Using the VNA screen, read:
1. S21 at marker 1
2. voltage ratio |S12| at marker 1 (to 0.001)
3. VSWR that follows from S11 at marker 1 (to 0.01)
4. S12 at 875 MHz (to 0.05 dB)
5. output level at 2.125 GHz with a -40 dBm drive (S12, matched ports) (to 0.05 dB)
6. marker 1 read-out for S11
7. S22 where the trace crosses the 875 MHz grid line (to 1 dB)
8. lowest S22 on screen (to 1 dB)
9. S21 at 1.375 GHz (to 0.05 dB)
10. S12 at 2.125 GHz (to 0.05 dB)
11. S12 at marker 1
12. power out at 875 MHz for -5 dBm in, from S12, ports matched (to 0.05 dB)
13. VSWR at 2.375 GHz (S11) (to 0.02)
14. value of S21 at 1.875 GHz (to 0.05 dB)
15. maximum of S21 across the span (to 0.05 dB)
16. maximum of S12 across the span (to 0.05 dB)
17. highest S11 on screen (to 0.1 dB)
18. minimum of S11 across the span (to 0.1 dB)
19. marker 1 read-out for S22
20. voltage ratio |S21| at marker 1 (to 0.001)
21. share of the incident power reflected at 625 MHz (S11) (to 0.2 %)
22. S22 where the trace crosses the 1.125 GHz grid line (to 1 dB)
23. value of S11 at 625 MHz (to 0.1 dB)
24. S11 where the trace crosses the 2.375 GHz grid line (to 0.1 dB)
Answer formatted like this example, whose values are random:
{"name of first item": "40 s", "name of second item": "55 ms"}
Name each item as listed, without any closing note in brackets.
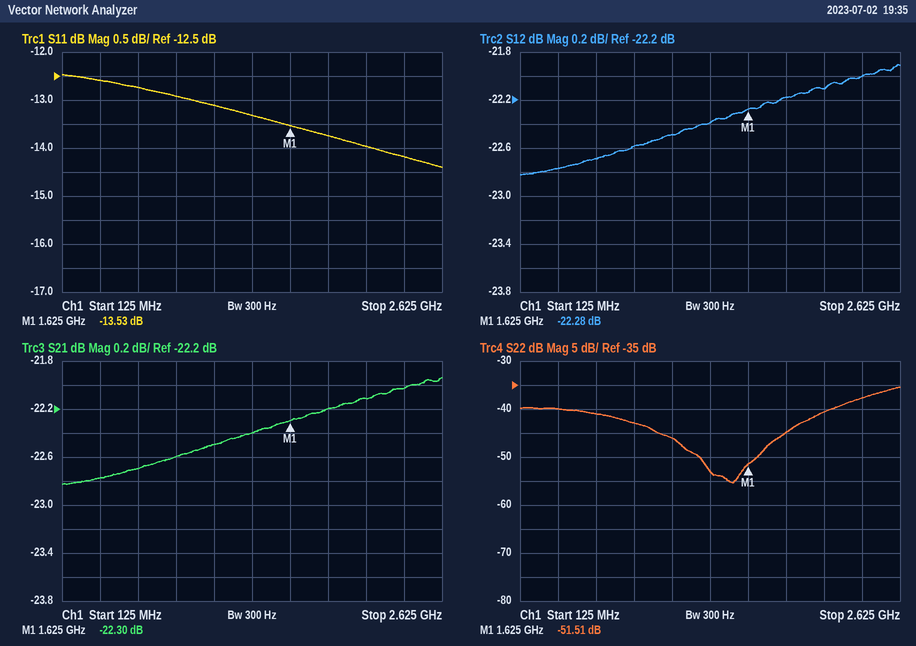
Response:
{"S21 at marker 1": "-22.30 dB", "voltage ratio |S12| at marker 1": "0.077", "VSWR that follows from S11 at marker 1": "1.53", "S12 at 875 MHz": "-22.60 dB", "output level at 2.125 GHz with a -40 dBm drive (S12, matched ports)": "-62.10 dBm", "marker 1 read-out for S11": "-13.53 dB", "S22 where the trace crosses the 875 MHz grid line": "-43 dB", "lowest S22 on screen": "-55 dB", "S21 at 1.375 GHz": "-22.40 dB", "S12 at 2.125 GHz": "-22.10 dB", "S12 at marker 1": "-22.28 dB", "power out at 875 MHz for -5 dBm in, from S12, ports matched": "-27.60 dBm", "VSWR at 2.375 GHz (S11)": "1.48", "value of S21 at 1.875 GHz": "-22.20 dB", "maximum of S21 across the span": "-21.95 dB", "maximum of S12 across the span": "-21.90 dB", "highest S11 on screen": "-12.5 dB", "minimum of S11 across the span": "-14.4 dB", "marker 1 read-out for S22": "-51.51 dB", "voltage ratio |S21| at marker 1": "0.077", "share of the incident power reflected at 625 MHz (S11)": "5.4 %", "S22 where the trace crosses the 1.125 GHz grid line": "-46 dB", "value of S11 at 625 MHz": "-12.7 dB", "S11 where the trace crosses the 2.375 GHz grid line": "-14.2 dB"}
